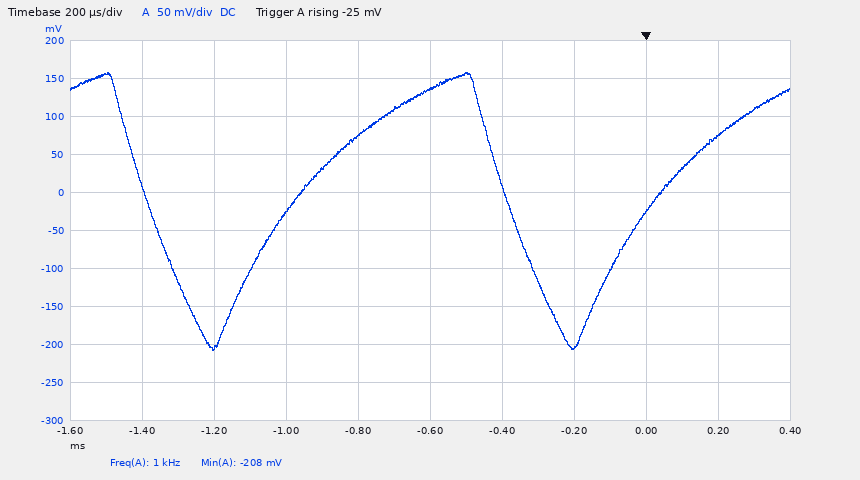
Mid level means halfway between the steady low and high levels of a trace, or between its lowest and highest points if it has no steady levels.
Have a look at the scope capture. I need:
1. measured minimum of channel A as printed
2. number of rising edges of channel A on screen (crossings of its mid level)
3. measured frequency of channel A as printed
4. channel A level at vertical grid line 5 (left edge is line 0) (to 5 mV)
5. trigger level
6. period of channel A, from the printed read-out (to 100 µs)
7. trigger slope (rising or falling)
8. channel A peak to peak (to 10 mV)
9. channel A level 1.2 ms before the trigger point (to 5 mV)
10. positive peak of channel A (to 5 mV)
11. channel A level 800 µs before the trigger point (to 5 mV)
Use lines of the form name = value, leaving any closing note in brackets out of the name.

measured minimum of channel A as printed = -208 mV
number of rising edges of channel A on screen = 2
measured frequency of channel A as printed = 1 kHz
channel A level at vertical grid line 5 (left edge is line 0) = 135 mV
trigger level = -25 mV
period of channel A, from the printed read-out = 1.0 ms
trigger slope = rising
channel A peak to peak = 370 mV
channel A level 1.2 ms before the trigger point = -205 mV
positive peak of channel A = 160 mV
channel A level 800 µs before the trigger point = 75 mV
